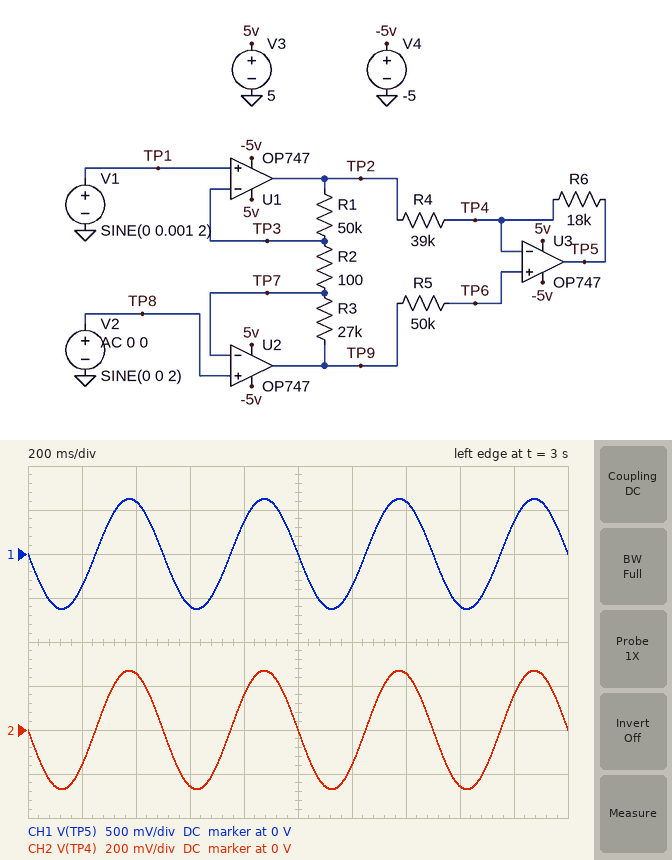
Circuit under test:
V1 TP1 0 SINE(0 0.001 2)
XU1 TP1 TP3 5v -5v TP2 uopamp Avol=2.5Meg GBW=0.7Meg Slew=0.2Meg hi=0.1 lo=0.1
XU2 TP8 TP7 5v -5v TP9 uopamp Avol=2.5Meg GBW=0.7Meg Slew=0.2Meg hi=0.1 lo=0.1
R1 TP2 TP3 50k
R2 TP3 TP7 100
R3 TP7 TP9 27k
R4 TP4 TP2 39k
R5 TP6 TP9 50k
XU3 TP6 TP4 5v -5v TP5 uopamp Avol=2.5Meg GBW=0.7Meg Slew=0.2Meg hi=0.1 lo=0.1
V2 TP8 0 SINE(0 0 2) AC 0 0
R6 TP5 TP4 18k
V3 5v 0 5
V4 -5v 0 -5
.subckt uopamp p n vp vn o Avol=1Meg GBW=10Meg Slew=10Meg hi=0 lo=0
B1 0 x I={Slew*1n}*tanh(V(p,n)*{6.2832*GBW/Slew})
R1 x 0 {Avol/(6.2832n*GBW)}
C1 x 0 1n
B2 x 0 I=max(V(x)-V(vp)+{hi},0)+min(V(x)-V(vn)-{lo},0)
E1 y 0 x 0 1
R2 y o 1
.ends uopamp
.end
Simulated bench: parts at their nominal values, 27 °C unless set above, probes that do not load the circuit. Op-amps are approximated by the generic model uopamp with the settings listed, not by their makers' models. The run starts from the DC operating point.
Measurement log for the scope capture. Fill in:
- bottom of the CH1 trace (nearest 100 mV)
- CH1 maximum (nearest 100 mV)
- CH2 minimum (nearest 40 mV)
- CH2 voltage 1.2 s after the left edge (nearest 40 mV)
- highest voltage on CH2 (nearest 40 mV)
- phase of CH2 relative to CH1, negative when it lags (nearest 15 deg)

-600 mV
600 mV
-280 mV
-160 mV
280 mV
0 deg
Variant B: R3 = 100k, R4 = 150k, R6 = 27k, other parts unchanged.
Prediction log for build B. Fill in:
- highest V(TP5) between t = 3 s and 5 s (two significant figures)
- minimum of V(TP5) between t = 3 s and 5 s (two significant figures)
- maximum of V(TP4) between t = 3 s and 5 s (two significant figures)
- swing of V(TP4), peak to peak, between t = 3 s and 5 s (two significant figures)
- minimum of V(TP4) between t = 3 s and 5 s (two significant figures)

1.3 V
-1.3 V
1.0 V
2.0 V
-1.0 V
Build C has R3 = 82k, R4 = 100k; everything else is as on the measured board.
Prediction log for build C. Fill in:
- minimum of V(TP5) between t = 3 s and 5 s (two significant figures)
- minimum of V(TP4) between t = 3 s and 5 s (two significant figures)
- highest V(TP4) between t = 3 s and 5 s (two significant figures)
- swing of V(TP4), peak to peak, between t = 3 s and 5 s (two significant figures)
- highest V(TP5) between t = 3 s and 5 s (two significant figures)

-1.1 V
-820 mV
820 mV
1.6 V
1.1 V
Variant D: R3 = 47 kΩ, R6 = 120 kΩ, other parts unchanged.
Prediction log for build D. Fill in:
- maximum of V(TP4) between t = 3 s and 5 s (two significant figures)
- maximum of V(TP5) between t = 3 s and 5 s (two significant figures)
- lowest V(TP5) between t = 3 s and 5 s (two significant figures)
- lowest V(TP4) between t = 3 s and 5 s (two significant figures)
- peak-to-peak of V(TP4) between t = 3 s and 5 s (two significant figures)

470 mV
3.5 V
-3.5 V
-470 mV
940 mV
